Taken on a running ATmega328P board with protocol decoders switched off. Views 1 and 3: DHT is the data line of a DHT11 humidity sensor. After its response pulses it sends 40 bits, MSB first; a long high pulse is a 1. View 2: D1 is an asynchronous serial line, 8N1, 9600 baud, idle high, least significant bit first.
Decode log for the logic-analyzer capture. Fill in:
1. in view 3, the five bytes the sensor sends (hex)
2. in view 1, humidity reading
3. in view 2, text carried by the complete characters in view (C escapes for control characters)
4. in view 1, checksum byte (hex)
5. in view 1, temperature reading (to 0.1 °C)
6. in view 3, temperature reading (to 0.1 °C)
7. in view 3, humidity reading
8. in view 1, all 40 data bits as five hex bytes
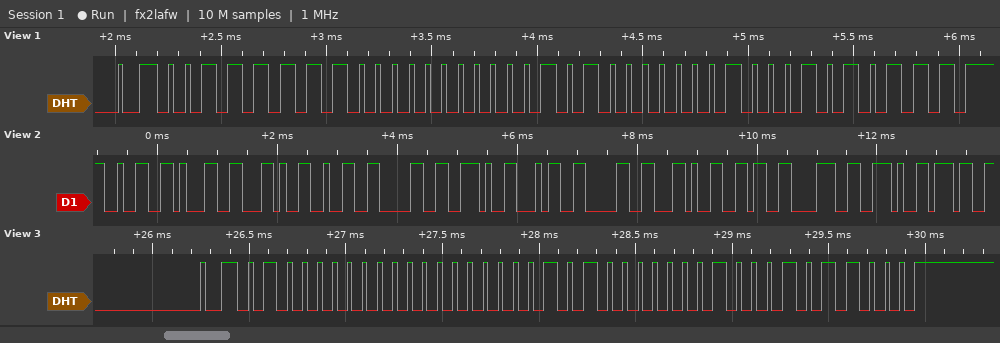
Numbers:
40 00 14 04 58
63 %
"21,20.40,68.7"
0x57
20.4 °C
20.4 °C
64 %
3F 00 14 04 57
